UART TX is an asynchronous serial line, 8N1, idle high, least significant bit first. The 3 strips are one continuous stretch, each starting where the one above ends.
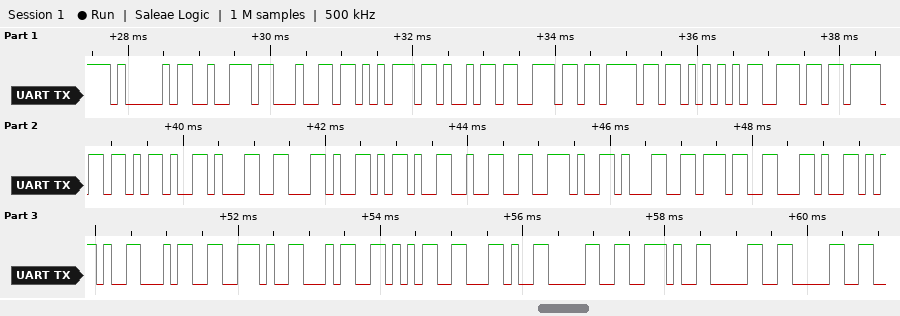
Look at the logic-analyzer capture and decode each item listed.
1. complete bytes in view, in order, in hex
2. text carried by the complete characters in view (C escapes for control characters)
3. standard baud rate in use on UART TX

0x41 0x72 0x64 0x75 0x69 0x6E 0x6F 0x55 0x6E 0x6F 0x2D 0x31 0x2C 0x2D 0x32 0x2E 0x31 0x37 0x2C 0x2D 0x34 0x2E 0x34 0x35 0x2C 0x30 0x2E 0x30 0x30
"ArduinoUno-1,-2.17,-4.45,0.00"
9600 baud
